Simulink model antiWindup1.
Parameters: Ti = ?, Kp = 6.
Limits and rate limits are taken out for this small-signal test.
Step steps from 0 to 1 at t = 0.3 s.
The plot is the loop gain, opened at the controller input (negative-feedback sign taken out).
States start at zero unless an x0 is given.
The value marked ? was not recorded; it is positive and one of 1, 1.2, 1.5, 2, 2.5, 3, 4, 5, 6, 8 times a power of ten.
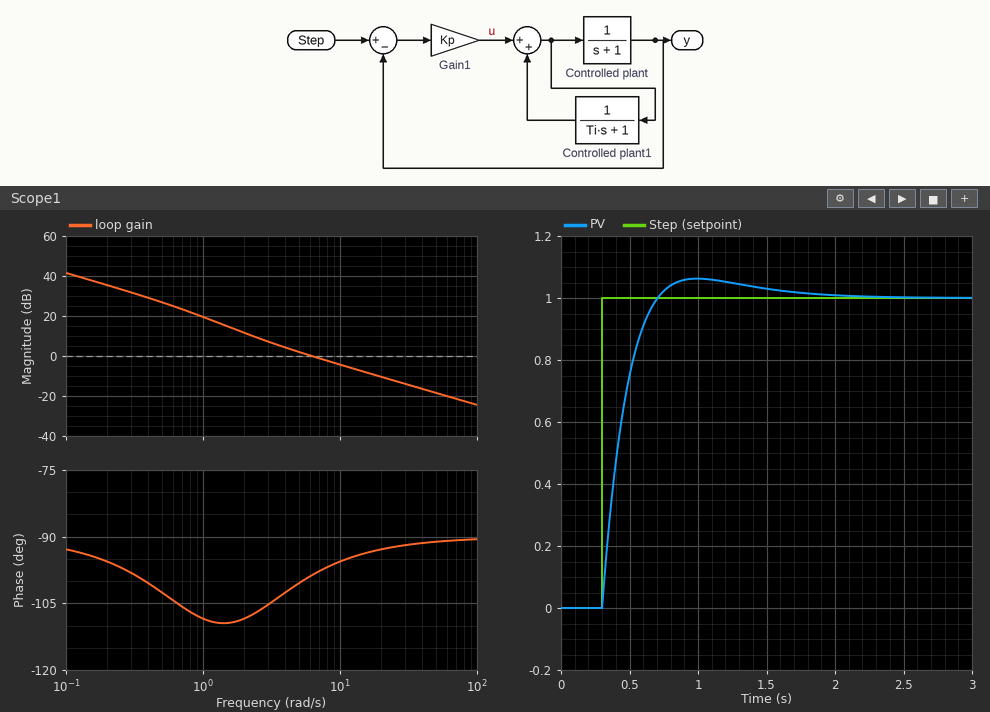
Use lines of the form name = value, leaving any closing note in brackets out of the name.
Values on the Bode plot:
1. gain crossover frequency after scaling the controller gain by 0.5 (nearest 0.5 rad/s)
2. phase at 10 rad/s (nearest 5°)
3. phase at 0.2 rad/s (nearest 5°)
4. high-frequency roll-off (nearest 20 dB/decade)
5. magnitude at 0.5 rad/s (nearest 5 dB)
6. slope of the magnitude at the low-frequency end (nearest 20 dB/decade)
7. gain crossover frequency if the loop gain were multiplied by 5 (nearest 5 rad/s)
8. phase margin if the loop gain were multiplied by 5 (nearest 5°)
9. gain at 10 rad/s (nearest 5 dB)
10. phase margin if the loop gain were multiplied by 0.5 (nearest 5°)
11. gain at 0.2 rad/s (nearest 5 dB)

gain crossover frequency after scaling the controller gain by 0.5 = 3.5 rad/s
phase at 10 rad/s = -95°
phase at 0.2 rad/s = -95°
high-frequency roll-off = -20 dB/decade
magnitude at 0.5 rad/s = 25 dB
slope of the magnitude at the low-frequency end = -20 dB/decade
gain crossover frequency if the loop gain were multiplied by 5 = 30 rad/s
phase margin if the loop gain were multiplied by 5 = 90°
gain at 10 rad/s = -5 dB
phase margin if the loop gain were multiplied by 0.5 = 75°
gain at 0.2 rad/s = 35 dB
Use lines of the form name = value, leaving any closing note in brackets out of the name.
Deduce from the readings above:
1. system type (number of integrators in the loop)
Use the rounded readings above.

system type = 1
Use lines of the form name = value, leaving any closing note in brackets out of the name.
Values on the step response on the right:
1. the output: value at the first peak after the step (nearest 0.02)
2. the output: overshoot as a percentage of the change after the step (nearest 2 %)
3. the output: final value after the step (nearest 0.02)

the output: value at the first peak after the step = 1.06
the output: overshoot as a percentage of the change after the step = 6 %
the output: final value after the step = 1.00
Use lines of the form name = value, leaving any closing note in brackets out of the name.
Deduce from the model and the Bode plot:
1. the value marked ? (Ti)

the value marked ? = 0.5
